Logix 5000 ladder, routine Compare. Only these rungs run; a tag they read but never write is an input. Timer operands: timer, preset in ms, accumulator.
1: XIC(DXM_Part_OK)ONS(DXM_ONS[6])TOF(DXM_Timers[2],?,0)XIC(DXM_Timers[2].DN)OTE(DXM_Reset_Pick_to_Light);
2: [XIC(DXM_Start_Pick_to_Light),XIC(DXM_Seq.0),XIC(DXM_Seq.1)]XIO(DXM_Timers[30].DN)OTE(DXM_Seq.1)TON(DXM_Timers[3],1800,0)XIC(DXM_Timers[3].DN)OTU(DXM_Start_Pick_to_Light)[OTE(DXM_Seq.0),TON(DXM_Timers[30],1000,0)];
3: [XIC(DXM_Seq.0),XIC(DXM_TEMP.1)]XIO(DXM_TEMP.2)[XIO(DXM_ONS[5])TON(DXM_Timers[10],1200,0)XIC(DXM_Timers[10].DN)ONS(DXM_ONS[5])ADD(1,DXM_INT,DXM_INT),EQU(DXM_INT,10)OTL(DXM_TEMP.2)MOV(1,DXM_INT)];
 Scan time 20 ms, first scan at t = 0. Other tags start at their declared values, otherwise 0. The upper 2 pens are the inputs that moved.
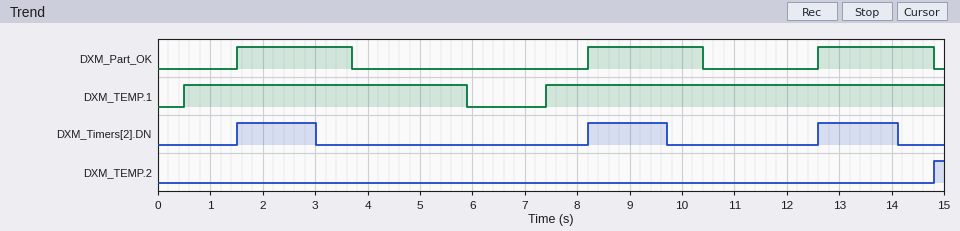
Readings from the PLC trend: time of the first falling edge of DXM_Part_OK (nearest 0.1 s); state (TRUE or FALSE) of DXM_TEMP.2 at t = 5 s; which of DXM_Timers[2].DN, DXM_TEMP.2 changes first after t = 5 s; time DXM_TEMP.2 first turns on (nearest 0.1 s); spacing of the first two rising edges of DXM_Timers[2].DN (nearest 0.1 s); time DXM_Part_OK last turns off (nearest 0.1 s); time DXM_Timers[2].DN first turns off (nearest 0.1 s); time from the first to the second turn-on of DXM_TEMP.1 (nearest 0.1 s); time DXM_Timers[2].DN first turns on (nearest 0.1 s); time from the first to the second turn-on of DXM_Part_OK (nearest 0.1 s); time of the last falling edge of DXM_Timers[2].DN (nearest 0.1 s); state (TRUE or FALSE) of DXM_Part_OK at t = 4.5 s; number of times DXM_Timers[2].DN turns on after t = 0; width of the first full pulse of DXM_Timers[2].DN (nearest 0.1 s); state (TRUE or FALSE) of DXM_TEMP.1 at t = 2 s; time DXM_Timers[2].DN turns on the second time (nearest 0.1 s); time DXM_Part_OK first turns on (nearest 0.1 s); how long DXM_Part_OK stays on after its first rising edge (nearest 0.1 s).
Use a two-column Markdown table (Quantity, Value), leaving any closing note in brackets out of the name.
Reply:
| Quantity | Value |
|---|---|
| time of the first falling edge of DXM_Part_OK | 3.7 s |
| state (TRUE or FALSE) of DXM_TEMP.2 at t = 5 s | FALSE |
| which of DXM_Timers[2].DN, DXM_TEMP.2 changes first after t = 5 s | DXM_Timers[2].DN |
| time DXM_TEMP.2 first turns on | 14.8 s |
| spacing of the first two rising edges of DXM_Timers[2].DN | 6.7 s |
| time DXM_Part_OK last turns off | 14.8 s |
| time DXM_Timers[2].DN first turns off | 3.0 s |
| time from the first to the second turn-on of DXM_TEMP.1 | 6.9 s |
| time DXM_Timers[2].DN first turns on | 1.5 s |
| time from the first to the second turn-on of DXM_Part_OK | 6.7 s |
| time of the last falling edge of DXM_Timers[2].DN | 14.1 s |
| state (TRUE or FALSE) of DXM_Part_OK at t = 4.5 s | FALSE |
| number of times DXM_Timers[2].DN turns on after t = 0 | 3 |
| width of the first full pulse of DXM_Timers[2].DN | 1.5 s |
| state (TRUE or FALSE) of DXM_TEMP.1 at t = 2 s | TRUE |
| time DXM_Timers[2].DN turns on the second time | 8.2 s |
| time DXM_Part_OK first turns on | 1.5 s |
| how long DXM_Part_OK stays on after its first rising edge | 2.2 s |
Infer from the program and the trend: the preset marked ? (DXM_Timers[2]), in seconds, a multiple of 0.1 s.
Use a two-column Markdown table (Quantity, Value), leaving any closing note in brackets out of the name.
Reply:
| Quantity | Value |
|---|---|
| the preset marked ? (DXM_Timers[2]), in seconds, a multiple of 0.1 s | 1.5 s |
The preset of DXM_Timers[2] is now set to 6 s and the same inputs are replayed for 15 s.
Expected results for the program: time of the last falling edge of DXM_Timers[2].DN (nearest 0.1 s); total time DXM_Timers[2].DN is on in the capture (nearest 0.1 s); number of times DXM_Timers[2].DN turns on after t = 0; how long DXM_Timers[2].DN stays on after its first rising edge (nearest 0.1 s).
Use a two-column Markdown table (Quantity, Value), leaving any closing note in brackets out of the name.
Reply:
| Quantity | Value |
|---|---|
| time of the last falling edge of DXM_Timers[2].DN | 7.5 s |
| total time DXM_Timers[2].DN is on in the capture | 12.8 s |
| number of times DXM_Timers[2].DN turns on after t = 0 | 2 |
| how long DXM_Timers[2].DN stays on after its first rising edge | 6.0 s |
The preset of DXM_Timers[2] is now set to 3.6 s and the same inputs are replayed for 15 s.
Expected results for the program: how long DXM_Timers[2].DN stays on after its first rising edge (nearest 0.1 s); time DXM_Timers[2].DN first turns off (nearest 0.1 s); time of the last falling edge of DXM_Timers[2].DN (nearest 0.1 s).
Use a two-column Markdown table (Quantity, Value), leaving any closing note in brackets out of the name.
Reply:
| Quantity | Value |
|---|---|
| how long DXM_Timers[2].DN stays on after its first rising edge | 3.6 s |
| time DXM_Timers[2].DN first turns off | 5.1 s |
| time of the last falling edge of DXM_Timers[2].DN | 11.8 s |
